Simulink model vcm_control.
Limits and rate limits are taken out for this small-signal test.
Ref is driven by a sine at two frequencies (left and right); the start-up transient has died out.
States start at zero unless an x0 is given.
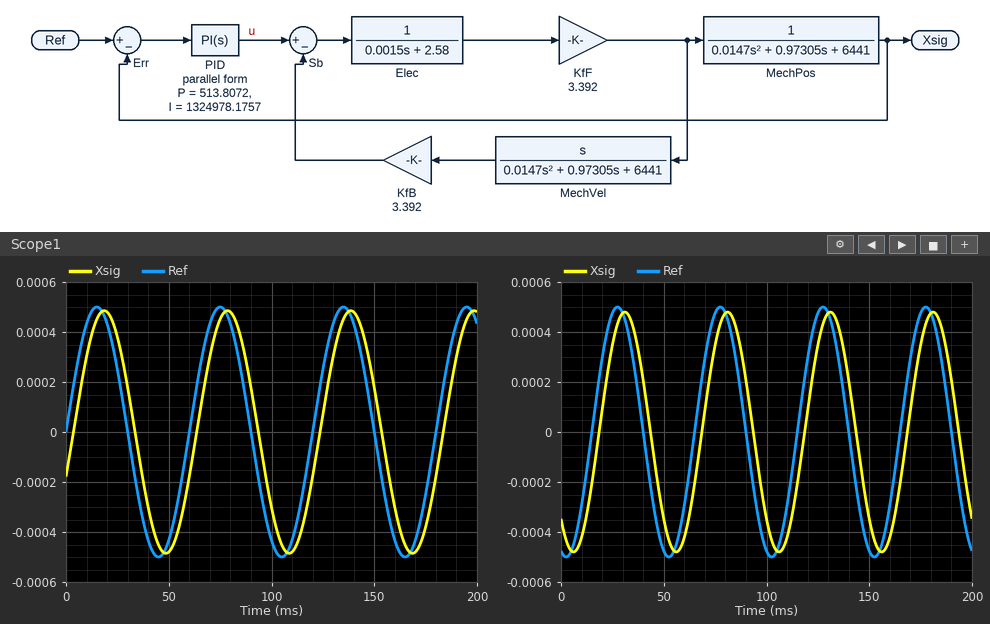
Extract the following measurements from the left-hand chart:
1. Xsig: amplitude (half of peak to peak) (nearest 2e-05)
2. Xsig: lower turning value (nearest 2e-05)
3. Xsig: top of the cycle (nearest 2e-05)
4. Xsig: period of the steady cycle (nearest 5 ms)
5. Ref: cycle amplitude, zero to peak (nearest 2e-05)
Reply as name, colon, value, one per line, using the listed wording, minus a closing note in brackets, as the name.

Xsig: amplitude (half of peak to peak): 0.00048
Xsig: lower turning value: -0.00048
Xsig: top of the cycle: 0.00048
Xsig: period of the steady cycle: 60 ms
Ref: cycle amplitude, zero to peak: 0.00050
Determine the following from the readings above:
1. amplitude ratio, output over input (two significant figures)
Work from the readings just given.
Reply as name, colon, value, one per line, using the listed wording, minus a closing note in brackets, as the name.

amplitude ratio, output over input: 0.96
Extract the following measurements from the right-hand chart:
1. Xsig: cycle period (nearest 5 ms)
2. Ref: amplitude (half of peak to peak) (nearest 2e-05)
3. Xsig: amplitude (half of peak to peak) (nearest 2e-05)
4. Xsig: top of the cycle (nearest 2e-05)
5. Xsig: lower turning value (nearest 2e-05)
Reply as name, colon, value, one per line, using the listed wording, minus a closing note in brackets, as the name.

Xsig: cycle period: 50 ms
Ref: amplitude (half of peak to peak): 0.00050
Xsig: amplitude (half of peak to peak): 0.00048
Xsig: top of the cycle: 0.00048
Xsig: lower turning value: -0.00048
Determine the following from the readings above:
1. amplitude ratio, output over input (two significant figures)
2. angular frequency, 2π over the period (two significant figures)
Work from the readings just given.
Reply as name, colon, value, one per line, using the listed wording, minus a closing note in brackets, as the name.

amplitude ratio, output over input: 0.96
angular frequency, 2π over the period: 0.13 rad/ms
